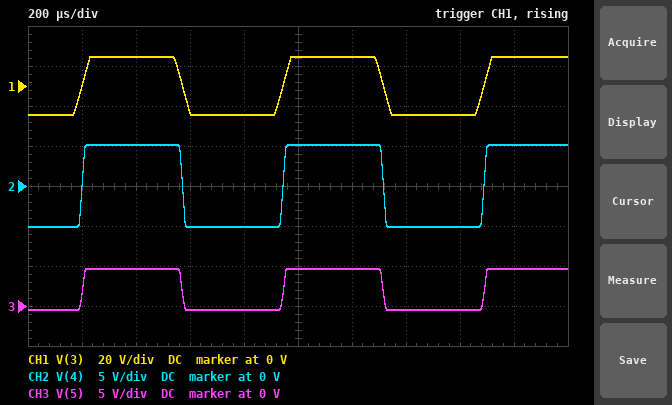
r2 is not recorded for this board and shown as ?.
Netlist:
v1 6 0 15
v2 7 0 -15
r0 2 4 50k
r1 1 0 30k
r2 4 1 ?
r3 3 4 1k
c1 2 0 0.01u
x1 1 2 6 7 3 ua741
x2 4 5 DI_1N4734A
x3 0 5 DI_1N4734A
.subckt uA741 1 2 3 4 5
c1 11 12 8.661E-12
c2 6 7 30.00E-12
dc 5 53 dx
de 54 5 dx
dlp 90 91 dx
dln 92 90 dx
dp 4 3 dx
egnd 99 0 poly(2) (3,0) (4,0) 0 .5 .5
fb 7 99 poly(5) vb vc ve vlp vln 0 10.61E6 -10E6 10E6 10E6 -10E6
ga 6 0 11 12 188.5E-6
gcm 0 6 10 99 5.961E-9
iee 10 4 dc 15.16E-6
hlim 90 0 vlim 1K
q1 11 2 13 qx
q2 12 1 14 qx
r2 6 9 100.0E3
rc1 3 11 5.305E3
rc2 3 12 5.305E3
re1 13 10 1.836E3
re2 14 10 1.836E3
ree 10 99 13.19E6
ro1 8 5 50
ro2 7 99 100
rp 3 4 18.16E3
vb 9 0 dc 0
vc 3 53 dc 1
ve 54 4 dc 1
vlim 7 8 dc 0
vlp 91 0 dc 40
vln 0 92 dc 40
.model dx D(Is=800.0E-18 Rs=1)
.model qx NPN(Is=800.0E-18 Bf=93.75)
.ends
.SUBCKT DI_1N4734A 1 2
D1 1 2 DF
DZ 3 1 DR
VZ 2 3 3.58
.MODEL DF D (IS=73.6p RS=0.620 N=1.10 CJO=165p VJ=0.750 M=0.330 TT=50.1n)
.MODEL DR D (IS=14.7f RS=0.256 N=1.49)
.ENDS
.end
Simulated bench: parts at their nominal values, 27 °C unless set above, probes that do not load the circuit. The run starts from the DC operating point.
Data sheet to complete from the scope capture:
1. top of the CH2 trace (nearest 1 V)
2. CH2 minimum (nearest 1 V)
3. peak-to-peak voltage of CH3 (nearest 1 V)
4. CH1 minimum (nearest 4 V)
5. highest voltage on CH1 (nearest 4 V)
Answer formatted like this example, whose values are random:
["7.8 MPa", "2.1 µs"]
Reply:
["5 V", "-5 V", "5 V", "-16 V", "16 V"]
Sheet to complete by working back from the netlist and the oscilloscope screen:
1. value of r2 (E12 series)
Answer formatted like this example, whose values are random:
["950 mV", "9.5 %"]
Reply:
["68 kΩ"]
